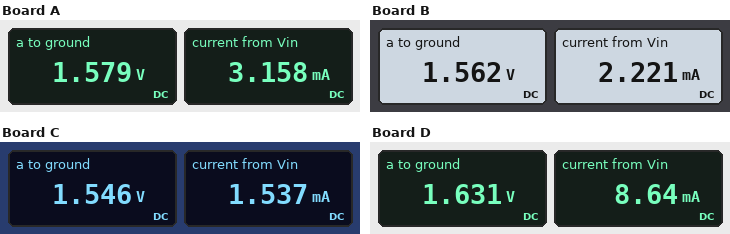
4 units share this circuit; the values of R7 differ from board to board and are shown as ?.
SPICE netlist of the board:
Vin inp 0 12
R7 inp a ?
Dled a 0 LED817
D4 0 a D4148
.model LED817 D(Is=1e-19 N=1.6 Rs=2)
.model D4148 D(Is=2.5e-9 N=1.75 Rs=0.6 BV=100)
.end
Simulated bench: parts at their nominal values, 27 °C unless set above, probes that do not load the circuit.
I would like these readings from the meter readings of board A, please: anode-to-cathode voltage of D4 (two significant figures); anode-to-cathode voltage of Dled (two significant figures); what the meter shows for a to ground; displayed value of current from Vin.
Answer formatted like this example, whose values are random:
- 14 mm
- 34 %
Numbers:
- -1.6 V
- 1.6 V
- 1.579 V
- 3.158 mA
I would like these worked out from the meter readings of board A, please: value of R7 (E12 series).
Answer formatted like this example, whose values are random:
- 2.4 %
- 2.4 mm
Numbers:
- 3.3 kΩ
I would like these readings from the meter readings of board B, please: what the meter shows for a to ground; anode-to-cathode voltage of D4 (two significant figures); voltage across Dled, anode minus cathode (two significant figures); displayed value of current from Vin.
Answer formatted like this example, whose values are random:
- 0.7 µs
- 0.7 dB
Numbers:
- 1.562 V
- -1.6 V
- 1.6 V
- 2.221 mA
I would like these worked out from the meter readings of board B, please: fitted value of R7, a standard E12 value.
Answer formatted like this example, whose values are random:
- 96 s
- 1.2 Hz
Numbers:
- 4.7 kΩ
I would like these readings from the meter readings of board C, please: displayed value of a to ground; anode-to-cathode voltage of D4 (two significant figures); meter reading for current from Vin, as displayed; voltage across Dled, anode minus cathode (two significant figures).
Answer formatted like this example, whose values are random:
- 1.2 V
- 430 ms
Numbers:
- 1.546 V
- -1.5 V
- 1.537 mA
- 1.5 V
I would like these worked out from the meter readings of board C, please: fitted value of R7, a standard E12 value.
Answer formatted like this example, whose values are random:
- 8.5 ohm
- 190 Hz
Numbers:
- 6.8 kΩ
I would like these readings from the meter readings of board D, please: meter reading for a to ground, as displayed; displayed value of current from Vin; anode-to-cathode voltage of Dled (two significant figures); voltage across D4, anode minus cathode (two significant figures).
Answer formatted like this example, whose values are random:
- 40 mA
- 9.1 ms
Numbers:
- 1.631 V
- 8.64 mA
- 1.6 V
- -1.6 V
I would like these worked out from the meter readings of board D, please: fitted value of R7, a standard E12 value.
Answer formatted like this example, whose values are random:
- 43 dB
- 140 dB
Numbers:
- 1.2 kΩ
